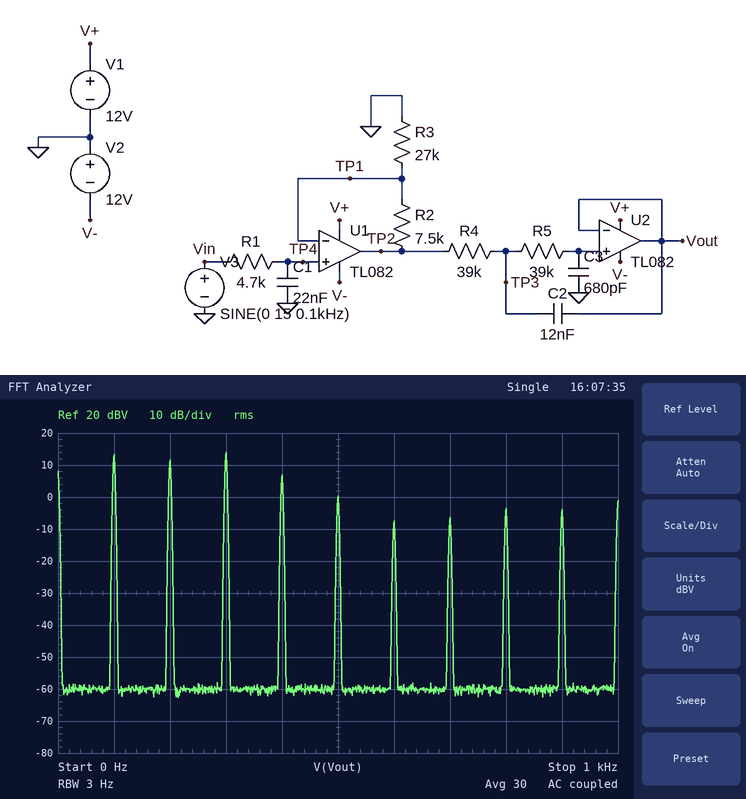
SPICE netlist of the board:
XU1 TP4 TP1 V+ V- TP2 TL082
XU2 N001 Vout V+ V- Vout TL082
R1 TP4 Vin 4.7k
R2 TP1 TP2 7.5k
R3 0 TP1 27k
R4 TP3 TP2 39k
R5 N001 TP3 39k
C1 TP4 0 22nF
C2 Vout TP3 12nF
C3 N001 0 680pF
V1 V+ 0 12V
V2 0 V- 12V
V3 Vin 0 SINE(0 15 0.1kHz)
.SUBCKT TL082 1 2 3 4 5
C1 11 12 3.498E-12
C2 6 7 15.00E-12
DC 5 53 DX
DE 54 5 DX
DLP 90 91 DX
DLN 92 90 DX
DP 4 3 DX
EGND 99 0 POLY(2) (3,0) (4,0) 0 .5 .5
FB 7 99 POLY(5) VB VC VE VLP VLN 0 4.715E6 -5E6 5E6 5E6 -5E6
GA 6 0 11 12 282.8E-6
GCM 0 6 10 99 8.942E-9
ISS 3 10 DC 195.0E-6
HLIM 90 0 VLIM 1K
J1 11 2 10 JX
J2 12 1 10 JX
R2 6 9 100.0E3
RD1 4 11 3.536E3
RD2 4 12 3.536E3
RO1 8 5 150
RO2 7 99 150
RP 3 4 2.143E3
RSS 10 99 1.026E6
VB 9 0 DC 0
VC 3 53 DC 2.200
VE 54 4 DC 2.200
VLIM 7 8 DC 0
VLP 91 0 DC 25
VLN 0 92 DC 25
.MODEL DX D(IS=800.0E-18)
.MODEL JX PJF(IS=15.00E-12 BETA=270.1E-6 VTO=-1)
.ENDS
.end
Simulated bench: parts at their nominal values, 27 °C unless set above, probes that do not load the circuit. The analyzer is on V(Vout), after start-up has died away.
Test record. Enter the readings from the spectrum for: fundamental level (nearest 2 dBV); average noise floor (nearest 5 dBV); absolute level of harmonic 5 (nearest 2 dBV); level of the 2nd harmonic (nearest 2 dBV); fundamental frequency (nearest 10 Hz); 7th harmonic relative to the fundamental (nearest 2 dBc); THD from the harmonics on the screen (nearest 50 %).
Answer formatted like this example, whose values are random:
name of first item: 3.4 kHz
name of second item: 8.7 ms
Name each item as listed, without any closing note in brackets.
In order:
fundamental level: 14 dBV
average noise floor: -60 dBV
absolute level of harmonic 5: 0 dBV
level of the 2nd harmonic: 12 dBV
fundamental frequency: 100 Hz
7th harmonic relative to the fundamental: -20 dBc
THD from the harmonics on the screen: 150 %
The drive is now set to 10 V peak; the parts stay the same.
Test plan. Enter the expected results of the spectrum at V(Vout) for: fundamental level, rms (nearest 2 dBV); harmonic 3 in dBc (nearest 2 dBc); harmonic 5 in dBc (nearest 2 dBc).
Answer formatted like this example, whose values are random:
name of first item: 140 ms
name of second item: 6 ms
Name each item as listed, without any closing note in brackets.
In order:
fundamental level, rms: 18 dBV
harmonic 3 in dBc: -22 dBc
harmonic 5 in dBc: -28 dBc
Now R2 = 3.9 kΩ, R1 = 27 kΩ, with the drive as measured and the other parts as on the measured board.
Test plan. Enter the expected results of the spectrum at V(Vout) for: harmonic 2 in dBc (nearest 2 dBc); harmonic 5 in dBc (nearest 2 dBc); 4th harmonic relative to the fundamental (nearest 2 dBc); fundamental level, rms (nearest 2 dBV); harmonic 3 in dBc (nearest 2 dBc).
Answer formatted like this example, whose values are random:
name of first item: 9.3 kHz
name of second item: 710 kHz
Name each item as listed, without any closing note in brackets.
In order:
harmonic 2 in dBc: -46 dBc
harmonic 5 in dBc: -38 dBc
4th harmonic relative to the fundamental: -50 dBc
fundamental level, rms: 18 dBV
harmonic 3 in dBc: -16 dBc
